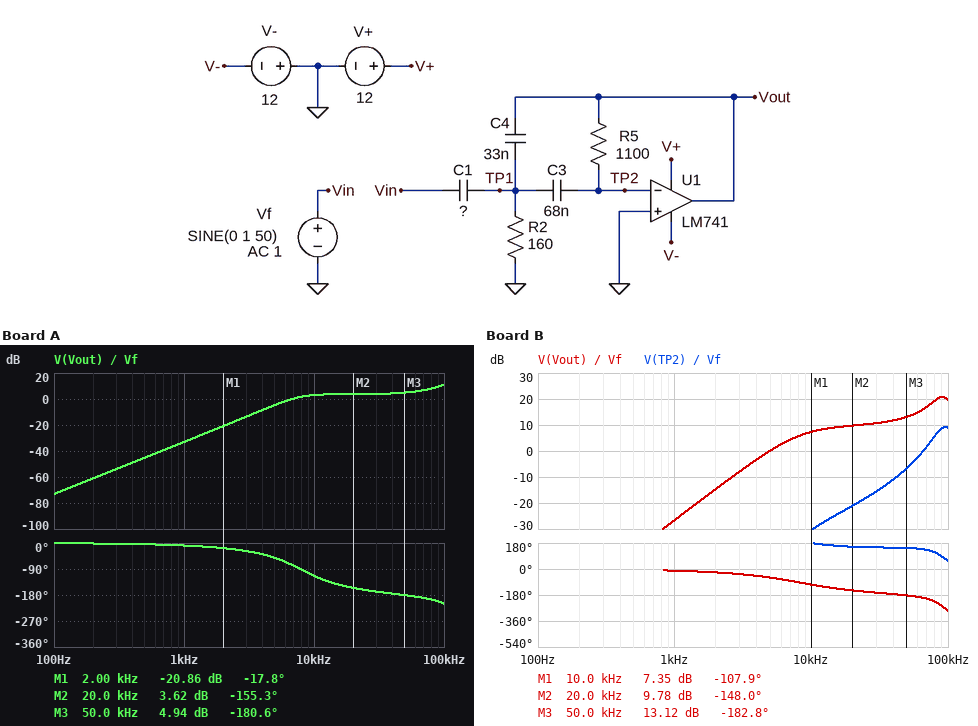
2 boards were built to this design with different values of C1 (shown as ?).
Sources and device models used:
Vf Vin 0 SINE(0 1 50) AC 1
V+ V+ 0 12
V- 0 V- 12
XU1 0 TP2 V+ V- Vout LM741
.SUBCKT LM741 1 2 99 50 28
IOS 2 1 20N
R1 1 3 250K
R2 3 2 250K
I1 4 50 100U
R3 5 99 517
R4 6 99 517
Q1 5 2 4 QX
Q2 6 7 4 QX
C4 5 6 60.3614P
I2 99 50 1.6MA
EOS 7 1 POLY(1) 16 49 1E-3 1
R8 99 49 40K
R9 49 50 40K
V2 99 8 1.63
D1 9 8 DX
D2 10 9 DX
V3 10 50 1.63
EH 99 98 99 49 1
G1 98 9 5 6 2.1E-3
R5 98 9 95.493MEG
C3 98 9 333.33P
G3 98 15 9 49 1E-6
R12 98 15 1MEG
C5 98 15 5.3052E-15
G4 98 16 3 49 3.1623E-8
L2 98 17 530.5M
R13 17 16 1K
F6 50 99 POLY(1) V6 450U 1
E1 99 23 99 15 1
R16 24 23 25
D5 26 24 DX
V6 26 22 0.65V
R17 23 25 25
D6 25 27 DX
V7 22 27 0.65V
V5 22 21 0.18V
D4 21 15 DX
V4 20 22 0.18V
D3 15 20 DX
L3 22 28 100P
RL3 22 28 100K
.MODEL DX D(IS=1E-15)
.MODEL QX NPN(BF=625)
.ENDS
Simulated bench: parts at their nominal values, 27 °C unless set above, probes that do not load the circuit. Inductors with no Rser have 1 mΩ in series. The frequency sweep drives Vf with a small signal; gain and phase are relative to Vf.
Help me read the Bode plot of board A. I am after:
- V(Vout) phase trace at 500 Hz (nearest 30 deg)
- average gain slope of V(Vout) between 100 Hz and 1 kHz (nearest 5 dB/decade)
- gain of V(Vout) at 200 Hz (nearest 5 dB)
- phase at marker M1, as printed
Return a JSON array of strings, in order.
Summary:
["0 deg", "40 dB/decade", "-60 dB", "-17.8 deg"]
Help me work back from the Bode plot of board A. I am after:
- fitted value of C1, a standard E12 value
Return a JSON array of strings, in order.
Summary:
["47 nF"]
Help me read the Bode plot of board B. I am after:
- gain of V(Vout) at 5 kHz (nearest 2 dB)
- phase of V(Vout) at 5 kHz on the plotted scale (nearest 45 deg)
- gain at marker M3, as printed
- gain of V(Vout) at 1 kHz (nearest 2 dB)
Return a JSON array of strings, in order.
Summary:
["0 dB", "-45 deg", "13.12 dB", "-26 dB"]
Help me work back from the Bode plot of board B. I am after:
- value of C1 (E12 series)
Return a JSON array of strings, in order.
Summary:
["100 nF"]
